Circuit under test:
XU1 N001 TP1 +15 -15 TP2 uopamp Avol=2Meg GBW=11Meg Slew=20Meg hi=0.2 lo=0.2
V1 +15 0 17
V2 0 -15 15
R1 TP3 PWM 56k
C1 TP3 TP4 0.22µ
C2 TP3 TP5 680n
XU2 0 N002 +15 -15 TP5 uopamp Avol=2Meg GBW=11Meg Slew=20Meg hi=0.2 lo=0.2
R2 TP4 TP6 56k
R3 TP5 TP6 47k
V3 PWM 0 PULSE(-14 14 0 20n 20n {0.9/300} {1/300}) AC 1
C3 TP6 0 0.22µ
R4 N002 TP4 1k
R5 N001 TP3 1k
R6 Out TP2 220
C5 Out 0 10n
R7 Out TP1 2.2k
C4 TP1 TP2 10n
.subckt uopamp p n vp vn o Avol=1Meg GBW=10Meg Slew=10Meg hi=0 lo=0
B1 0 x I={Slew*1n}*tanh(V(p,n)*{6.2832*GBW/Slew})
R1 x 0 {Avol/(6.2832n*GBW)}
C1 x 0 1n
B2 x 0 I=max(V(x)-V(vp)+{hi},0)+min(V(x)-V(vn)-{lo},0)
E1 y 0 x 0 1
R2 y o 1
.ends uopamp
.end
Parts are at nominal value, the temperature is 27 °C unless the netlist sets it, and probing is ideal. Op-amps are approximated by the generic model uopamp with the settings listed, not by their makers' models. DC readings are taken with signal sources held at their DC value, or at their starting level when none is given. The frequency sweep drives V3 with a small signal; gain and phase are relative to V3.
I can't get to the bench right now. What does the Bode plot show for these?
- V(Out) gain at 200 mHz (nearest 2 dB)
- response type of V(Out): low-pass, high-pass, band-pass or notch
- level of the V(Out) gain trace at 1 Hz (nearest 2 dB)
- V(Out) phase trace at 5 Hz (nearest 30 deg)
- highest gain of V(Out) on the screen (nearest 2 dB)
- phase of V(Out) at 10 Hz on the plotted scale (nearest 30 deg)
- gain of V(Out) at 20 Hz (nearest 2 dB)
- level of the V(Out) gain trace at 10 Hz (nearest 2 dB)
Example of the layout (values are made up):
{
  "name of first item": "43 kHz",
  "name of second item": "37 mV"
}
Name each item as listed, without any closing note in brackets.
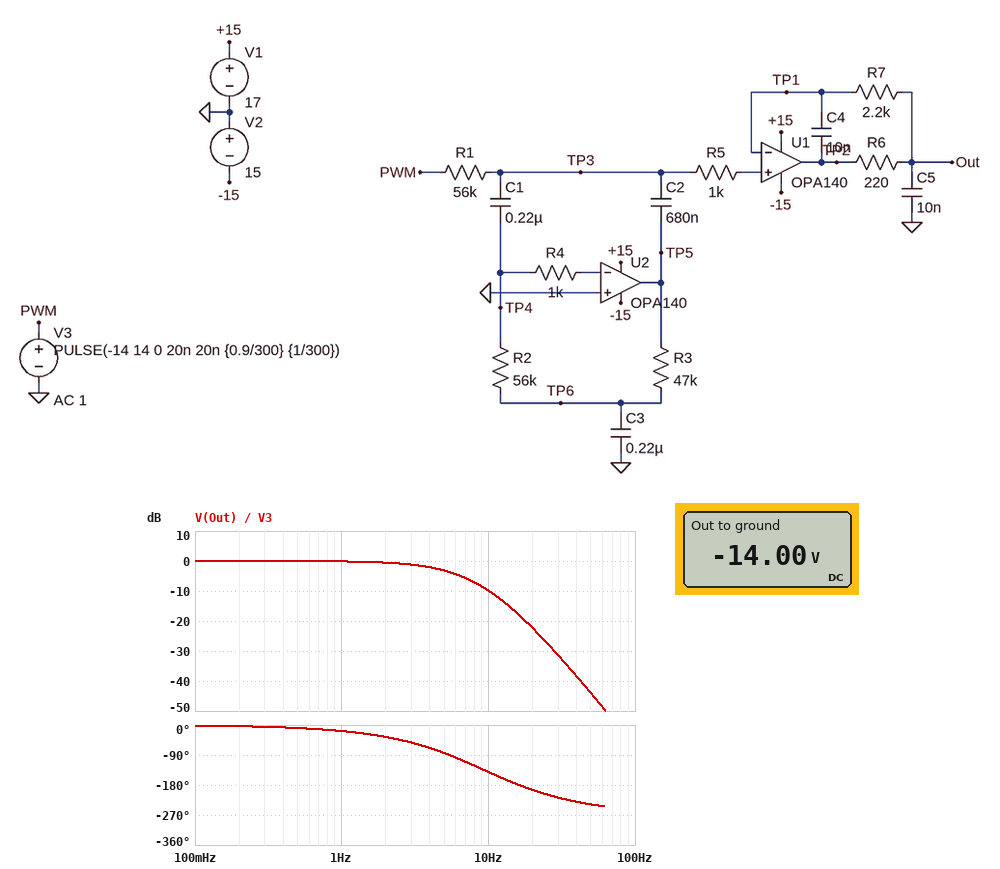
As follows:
{
  "V(Out) gain at 200 mHz": "0 dB",
  "response type of V(Out): low-pass, high-pass, band-pass or notch": "low-pass",
  "level of the V(Out) gain trace at 1 Hz": "0 dB",
  "V(Out) phase trace at 5 Hz": "-90 deg",
  "highest gain of V(Out) on the screen": "0 dB",
  "phase of V(Out) at 10 Hz on the plotted scale": "-150 deg",
  "gain of V(Out) at 20 Hz": "-22 dB",
  "level of the V(Out) gain trace at 10 Hz": "-10 dB"
}
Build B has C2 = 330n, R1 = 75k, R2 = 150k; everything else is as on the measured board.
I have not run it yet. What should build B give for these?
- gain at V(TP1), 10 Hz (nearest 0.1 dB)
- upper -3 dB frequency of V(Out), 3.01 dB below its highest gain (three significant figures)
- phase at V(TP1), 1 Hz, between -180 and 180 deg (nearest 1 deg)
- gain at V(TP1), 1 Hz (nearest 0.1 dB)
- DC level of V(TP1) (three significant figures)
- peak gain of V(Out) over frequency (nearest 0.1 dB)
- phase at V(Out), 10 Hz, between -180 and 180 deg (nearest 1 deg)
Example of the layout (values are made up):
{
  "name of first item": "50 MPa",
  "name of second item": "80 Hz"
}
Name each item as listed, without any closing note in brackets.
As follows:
{
  "gain at V(TP1), 10 Hz": "-10.3 dB",
  "upper -3 dB frequency of V(Out), 3.01 dB below its highest gain": "6.43 Hz",
  "phase at V(TP1), 1 Hz, between -180 and 180 deg": "-15 deg",
  "gain at V(TP1), 1 Hz": "0.1 dB",
  "DC level of V(TP1)": "-14.0 V",
  "peak gain of V(Out) over frequency": "0.5 dB",
  "phase at V(Out), 10 Hz, between -180 and 180 deg": "-171 deg"
}
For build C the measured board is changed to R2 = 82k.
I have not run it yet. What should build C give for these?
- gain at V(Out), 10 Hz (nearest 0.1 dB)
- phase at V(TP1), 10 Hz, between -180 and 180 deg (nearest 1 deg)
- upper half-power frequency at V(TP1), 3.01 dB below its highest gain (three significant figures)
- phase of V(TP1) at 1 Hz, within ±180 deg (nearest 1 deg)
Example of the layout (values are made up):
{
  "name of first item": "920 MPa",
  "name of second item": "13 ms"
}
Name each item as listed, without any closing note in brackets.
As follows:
{
  "gain at V(Out), 10 Hz": "-11.0 dB",
  "phase at V(TP1), 10 Hz, between -180 and 180 deg": "-157 deg",
  "upper half-power frequency at V(TP1), 3.01 dB below its highest gain": "5.23 Hz",
  "phase of V(TP1) at 1 Hz, within ±180 deg": "-18 deg"
}
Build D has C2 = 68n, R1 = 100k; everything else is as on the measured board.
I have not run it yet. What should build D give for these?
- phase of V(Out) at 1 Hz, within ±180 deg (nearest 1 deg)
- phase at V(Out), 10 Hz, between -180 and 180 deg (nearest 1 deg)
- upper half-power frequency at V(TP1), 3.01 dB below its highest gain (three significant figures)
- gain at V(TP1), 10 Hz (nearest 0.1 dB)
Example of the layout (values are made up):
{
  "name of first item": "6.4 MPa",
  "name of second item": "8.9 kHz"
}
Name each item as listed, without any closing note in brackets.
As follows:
{
  "phase of V(Out) at 1 Hz, within ±180 deg": "-10 deg",
  "phase at V(Out), 10 Hz, between -180 and 180 deg": "-76 deg",
  "upper half-power frequency at V(TP1), 3.01 dB below its highest gain": "7.35 Hz",
  "gain at V(TP1), 10 Hz": "-4.3 dB"
}
